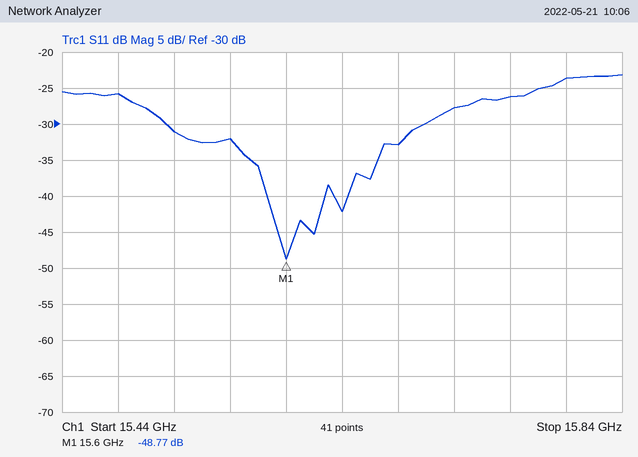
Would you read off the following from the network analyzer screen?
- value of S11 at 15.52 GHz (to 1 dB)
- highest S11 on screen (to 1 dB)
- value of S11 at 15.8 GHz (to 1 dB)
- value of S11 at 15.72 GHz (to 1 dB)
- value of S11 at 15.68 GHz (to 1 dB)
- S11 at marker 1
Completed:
-31 dB
-23 dB
-24 dB
-28 dB
-33 dB
-48.77 dB
